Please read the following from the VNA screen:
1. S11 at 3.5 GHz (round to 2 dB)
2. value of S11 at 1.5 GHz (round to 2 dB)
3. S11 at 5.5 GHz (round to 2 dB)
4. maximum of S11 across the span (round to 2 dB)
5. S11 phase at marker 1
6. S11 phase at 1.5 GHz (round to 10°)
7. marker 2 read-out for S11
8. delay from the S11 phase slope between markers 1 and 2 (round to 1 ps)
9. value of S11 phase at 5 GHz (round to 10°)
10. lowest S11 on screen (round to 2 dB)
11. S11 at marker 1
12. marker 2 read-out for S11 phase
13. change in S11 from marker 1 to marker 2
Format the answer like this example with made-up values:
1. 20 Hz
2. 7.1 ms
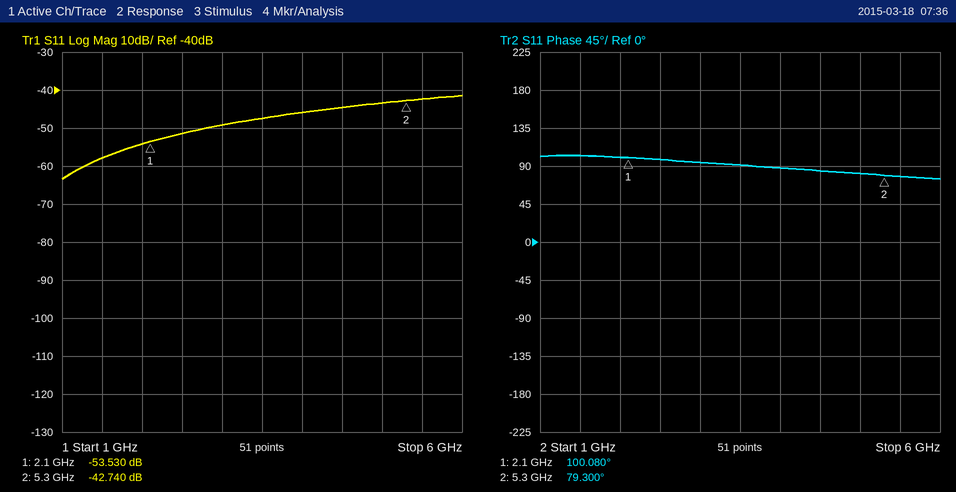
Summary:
1. -48 dB
2. -58 dB
3. -42 dB
4. -42 dB
5. 100.080°
6. 100°
7. -42.740 dB
8. 18 ps
9. 80°
10. -64 dB
11. -53.530 dB
12. 79.300°
13. 10.790 dB
